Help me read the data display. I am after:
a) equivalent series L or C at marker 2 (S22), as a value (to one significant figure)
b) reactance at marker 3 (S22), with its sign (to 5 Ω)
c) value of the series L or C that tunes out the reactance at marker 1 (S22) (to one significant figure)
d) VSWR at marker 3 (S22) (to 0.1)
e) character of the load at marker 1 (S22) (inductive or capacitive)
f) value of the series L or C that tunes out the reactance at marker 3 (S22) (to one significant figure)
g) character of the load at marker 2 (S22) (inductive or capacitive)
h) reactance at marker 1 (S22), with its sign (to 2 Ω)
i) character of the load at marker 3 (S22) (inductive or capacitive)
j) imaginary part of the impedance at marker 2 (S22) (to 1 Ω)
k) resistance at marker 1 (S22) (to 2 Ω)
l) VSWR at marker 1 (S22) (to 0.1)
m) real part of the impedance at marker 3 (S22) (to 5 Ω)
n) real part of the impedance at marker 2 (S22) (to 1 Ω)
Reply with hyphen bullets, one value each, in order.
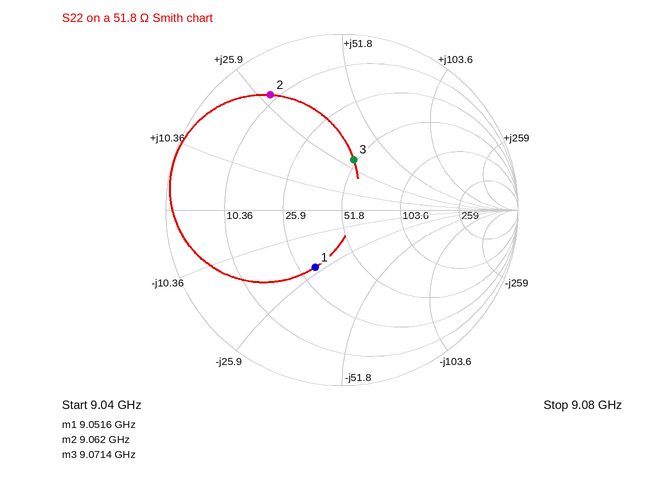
- 500 pH
- +30 Ω
- 400 pH
- 1.8
- capacitive
- 600 fF
- inductive
- -24 Ω
- inductive
- +28 Ω
- 32 Ω
- 2.1
- 50 Ω
- 9 Ω
